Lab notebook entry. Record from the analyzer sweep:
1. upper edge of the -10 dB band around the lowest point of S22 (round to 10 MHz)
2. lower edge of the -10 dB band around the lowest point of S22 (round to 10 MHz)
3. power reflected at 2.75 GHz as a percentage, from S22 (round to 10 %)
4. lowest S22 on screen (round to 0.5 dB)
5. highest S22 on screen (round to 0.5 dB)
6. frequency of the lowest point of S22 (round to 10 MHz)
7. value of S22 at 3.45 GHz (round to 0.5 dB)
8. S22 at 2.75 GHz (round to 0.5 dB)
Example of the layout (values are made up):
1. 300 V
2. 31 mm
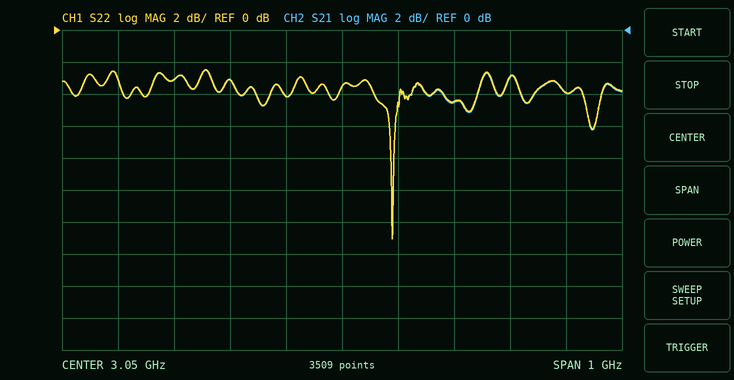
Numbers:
1. 3.14 GHz
2. 3.14 GHz
3. 50 %
4. -13.0 dB
5. -2.5 dB
6. 3.14 GHz
7. -4.0 dB
8. -3.0 dB
